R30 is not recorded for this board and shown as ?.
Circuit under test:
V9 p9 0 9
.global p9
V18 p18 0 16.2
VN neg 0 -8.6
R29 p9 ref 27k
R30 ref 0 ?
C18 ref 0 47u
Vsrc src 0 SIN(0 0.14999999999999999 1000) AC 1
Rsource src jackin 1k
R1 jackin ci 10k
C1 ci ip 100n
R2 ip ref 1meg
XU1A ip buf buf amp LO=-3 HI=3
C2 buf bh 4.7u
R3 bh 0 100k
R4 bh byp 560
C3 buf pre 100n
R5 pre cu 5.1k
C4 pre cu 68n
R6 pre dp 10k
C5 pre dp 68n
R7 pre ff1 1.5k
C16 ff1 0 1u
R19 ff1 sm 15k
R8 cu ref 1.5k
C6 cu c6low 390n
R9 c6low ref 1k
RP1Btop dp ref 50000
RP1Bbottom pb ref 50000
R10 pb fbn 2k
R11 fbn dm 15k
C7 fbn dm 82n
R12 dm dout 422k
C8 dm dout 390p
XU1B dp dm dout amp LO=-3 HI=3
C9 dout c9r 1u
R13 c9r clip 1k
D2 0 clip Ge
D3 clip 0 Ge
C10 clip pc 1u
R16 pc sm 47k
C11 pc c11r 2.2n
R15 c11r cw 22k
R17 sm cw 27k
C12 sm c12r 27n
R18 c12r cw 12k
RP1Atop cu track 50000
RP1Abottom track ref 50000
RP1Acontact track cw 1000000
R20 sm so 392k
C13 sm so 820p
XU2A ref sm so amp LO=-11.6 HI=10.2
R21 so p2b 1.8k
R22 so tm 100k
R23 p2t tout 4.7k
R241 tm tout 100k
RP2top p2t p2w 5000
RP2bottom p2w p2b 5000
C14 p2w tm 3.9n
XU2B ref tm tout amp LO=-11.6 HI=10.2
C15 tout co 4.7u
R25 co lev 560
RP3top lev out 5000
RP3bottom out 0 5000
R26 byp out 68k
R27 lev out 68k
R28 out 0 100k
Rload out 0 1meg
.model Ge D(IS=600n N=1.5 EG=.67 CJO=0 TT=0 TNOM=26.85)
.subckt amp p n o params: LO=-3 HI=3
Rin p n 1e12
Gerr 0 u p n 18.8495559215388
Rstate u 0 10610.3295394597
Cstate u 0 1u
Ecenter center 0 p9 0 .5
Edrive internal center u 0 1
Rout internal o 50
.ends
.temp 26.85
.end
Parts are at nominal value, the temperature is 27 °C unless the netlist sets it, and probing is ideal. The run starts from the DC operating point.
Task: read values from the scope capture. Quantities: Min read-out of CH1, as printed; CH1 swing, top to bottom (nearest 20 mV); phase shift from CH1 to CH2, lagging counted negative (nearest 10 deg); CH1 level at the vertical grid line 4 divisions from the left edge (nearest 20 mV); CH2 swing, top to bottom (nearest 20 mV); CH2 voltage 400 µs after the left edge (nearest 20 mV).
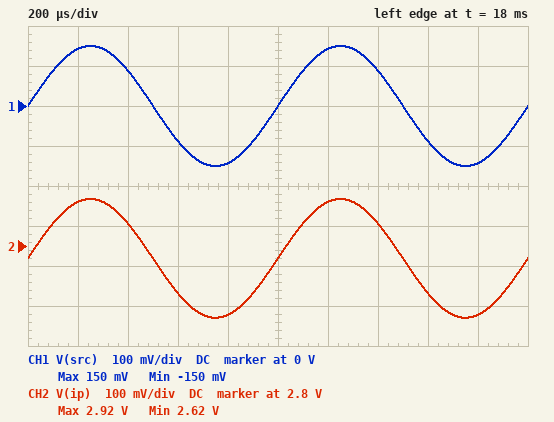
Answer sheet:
-150 mV
300 mV
0 deg
-140 mV
300 mV
2.86 V
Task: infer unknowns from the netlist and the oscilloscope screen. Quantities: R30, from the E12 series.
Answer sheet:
12 kΩ
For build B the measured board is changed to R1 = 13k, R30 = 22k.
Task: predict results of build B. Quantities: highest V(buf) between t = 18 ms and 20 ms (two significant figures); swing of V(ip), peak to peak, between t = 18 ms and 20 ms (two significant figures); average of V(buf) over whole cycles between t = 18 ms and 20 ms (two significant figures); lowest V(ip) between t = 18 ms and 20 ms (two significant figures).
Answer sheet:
4.2 V
300 mV
4.0 V
3.9 V
